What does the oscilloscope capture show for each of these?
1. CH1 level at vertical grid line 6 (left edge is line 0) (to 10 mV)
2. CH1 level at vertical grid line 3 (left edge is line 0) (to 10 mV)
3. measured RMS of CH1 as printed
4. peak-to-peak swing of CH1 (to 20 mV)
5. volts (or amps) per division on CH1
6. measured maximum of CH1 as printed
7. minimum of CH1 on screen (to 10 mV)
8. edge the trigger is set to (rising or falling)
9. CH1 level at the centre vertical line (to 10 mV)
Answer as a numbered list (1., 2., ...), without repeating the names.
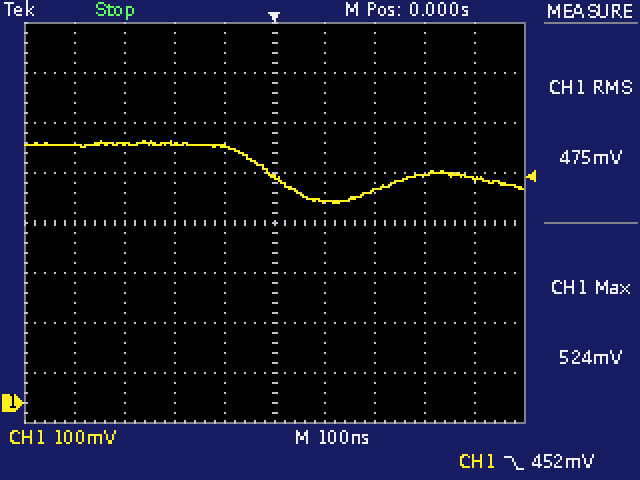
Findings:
1. 400 mV
2. 520 mV
3. 475 mV
4. 120 mV
5. 100 mV
6. 524 mV
7. 400 mV
8. falling
9. 450 mV
